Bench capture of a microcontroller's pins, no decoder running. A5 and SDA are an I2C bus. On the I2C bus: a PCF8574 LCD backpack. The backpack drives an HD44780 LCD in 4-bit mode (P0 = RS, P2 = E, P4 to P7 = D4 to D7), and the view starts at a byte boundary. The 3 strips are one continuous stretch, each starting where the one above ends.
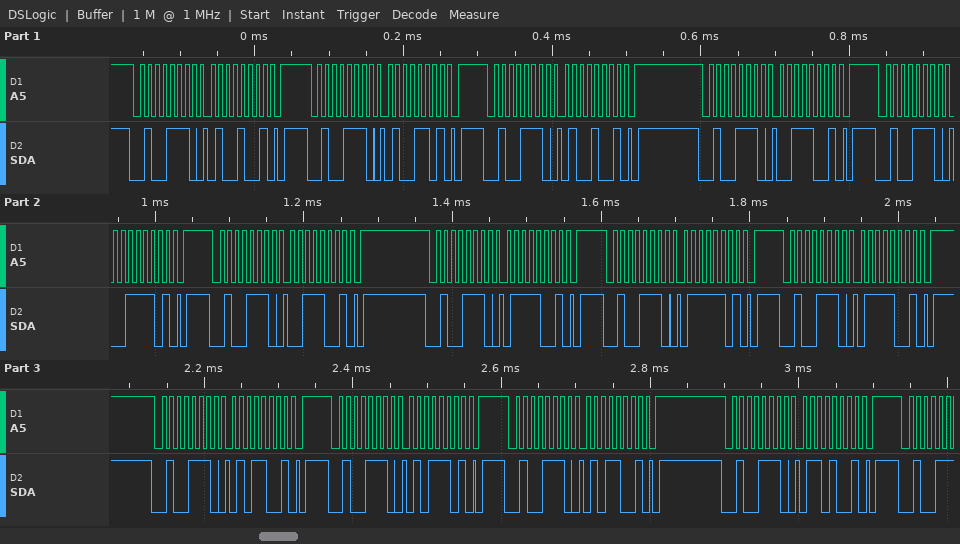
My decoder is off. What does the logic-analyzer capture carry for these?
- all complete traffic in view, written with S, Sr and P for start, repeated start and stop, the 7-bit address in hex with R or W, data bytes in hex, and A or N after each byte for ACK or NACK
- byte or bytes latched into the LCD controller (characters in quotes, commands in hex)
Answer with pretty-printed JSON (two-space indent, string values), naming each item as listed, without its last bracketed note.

{
  "all complete traffic in view, written with S, Sr and P for start, repeated start and stop, the 7-bit address in hex with R or W, data bytes in hex, and A or N after each byte for ACK or NACK": "S 27W A 49 A P S 27W A 4D A P S 27W A 49 A P S 27W A 39 A P S 27W A 3D A P S 27W A 39 A P S 27W A 79 A P S 27W A 7D A P S 27W A 79 A P S 27W A 59 A P S 27W A 5D A P S 27W A 59 A P S 27W A 69 A P",
  "byte or bytes latched into the LCD controller": "'C' 'u'"
}
